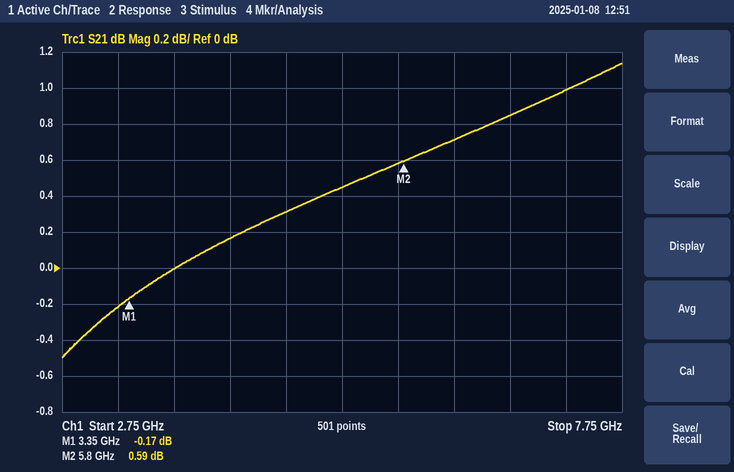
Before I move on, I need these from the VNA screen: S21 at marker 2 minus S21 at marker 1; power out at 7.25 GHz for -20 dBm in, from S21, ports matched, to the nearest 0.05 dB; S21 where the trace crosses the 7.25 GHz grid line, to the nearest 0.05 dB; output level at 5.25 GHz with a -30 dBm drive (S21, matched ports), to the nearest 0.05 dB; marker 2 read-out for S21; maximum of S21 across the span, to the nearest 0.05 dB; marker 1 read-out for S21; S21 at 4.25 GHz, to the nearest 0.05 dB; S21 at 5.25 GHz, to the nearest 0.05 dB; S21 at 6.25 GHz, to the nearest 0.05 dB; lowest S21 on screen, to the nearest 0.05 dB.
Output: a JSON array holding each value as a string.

["0.76 dB", "-19.00 dBm", "1.00 dB", "-29.55 dBm", "0.59 dB", "1.15 dB", "-0.17 dB", "0.15 dB", "0.45 dB", "0.70 dB", "-0.50 dB"]
